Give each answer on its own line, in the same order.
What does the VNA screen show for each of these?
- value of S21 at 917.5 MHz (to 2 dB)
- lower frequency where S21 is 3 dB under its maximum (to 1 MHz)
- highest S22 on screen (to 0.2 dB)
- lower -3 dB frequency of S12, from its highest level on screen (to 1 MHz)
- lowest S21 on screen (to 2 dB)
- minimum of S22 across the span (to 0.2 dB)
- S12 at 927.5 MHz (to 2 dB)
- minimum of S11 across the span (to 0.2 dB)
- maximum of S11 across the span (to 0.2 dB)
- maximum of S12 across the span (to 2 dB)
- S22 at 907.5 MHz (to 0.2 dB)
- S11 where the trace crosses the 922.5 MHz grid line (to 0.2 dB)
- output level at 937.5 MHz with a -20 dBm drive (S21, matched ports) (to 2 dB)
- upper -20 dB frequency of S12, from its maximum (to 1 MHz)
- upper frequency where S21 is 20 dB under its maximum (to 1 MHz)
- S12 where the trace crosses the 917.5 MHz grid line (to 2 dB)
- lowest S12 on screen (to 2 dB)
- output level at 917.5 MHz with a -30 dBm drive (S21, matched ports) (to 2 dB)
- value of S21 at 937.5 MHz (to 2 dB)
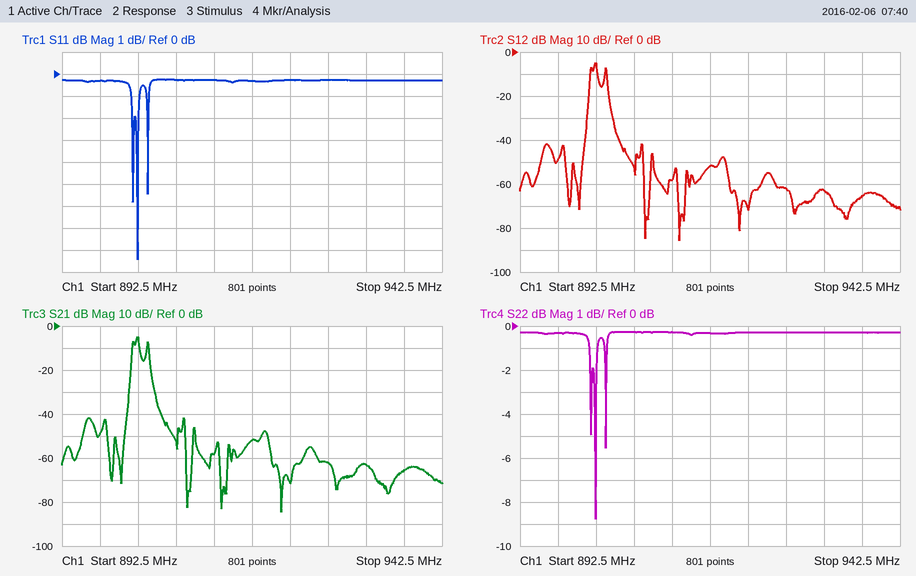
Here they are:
-52 dB
902 MHz
-0.2 dB
902 MHz
-84 dB
-8.8 dB
-62 dB
-8.4 dB
-0.2 dB
-4 dB
-0.2 dB
-0.2 dB
-86 dBm
904 MHz
904 MHz
-52 dB
-86 dB
-82 dBm
-66 dB
